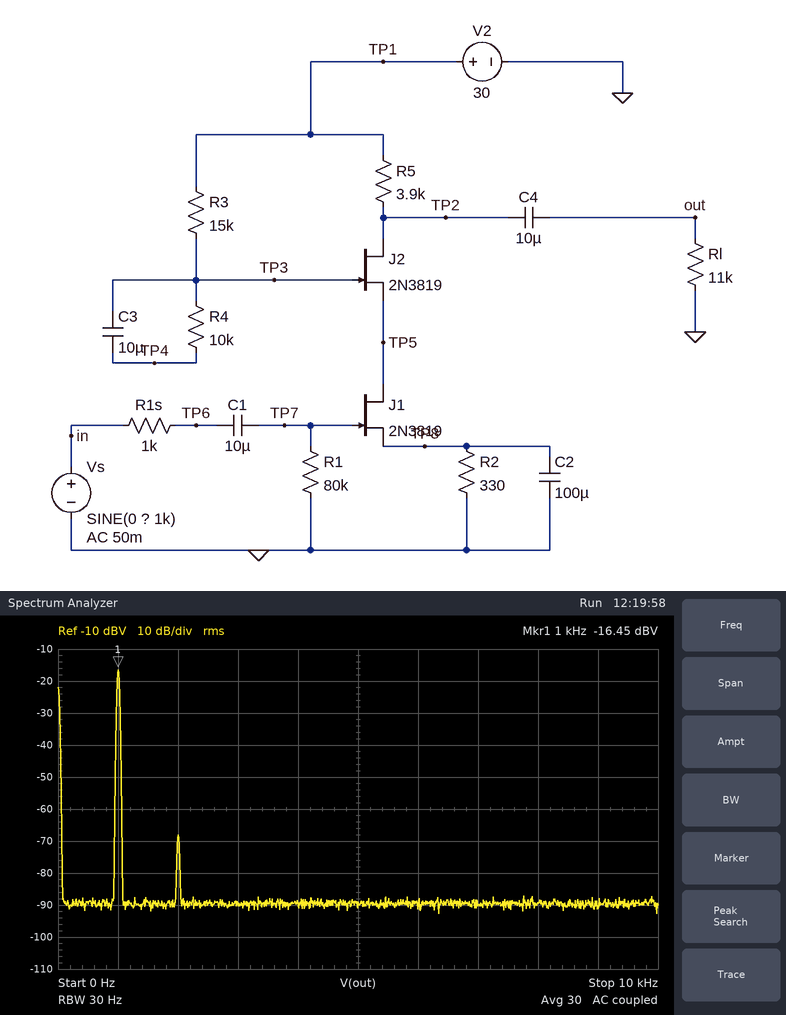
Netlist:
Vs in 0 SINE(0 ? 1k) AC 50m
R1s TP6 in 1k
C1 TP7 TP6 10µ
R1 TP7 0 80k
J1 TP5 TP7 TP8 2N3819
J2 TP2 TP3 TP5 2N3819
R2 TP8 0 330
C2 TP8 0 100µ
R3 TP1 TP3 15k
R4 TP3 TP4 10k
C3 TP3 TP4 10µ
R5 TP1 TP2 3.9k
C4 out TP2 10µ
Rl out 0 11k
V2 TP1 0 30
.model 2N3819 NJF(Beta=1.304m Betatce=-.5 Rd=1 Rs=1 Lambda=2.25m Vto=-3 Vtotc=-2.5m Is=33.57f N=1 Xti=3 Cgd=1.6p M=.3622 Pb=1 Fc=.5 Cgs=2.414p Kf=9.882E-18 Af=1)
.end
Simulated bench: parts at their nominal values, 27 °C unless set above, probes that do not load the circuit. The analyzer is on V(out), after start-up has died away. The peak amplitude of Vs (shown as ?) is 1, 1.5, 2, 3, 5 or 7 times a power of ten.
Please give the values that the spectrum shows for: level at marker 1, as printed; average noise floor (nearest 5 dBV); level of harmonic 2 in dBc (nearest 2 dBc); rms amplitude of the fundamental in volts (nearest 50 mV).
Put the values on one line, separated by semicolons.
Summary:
-16.45 dBV; -90 dBV; -52 dBc; 150 mV
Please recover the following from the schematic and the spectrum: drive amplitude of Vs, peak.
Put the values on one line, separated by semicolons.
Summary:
20 mV
